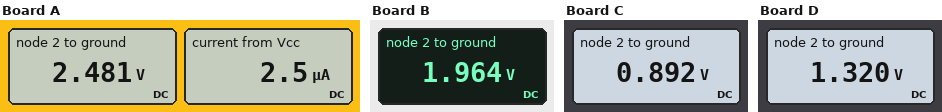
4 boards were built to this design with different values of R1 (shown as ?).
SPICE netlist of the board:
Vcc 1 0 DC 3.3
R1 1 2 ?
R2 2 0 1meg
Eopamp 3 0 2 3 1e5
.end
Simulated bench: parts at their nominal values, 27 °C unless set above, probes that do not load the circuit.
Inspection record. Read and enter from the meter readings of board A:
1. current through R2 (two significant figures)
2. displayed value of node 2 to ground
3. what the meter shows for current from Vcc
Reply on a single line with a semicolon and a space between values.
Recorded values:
2.5 µA; 2.481 V; 2.5 µA
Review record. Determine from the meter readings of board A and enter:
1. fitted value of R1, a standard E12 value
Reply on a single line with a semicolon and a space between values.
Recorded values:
330 kΩ
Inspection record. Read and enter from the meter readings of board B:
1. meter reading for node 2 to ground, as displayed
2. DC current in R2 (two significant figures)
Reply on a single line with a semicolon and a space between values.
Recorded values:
1.964 V; 2.0 µA
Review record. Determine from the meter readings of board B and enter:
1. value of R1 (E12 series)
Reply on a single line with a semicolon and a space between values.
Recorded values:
680 kΩ
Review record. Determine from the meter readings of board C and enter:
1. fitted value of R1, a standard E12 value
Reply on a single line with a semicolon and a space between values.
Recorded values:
2.7 MΩ
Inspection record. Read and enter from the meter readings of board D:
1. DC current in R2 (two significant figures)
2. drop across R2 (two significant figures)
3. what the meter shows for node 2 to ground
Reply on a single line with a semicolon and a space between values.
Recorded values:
1.3 µA; 1.3 V; 1.320 V
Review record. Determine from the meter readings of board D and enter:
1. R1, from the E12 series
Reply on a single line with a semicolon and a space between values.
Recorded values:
1.5 MΩ
